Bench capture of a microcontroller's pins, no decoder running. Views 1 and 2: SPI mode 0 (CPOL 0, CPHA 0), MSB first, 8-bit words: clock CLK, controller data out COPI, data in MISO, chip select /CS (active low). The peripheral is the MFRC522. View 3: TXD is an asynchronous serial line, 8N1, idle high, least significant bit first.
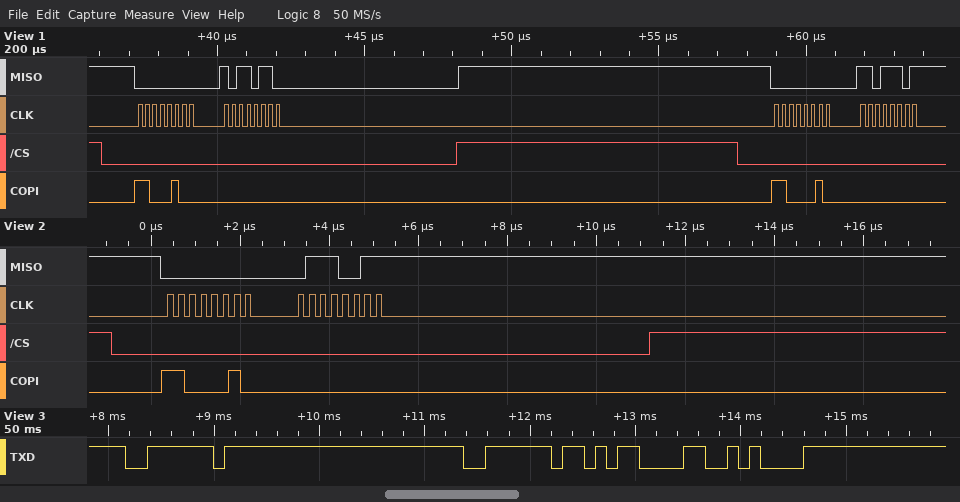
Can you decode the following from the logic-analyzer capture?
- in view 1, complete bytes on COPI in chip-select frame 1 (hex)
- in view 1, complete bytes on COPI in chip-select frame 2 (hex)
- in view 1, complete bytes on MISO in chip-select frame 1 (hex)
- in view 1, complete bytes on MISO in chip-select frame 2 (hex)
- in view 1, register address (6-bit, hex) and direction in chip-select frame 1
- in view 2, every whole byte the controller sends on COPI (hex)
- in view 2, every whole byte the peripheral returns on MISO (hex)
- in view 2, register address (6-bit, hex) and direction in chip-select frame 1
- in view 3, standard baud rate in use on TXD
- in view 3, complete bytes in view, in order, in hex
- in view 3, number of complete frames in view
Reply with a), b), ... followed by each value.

a) C4 00
b) C2 00
c) 00 B6
d) 00 DD
e) 0x22 read
f) C2 00
g) 00 73
h) 0x21 read
i) 9600 baud
j) 0x7E 0x7E 0x0D 0x0A
k) 4
